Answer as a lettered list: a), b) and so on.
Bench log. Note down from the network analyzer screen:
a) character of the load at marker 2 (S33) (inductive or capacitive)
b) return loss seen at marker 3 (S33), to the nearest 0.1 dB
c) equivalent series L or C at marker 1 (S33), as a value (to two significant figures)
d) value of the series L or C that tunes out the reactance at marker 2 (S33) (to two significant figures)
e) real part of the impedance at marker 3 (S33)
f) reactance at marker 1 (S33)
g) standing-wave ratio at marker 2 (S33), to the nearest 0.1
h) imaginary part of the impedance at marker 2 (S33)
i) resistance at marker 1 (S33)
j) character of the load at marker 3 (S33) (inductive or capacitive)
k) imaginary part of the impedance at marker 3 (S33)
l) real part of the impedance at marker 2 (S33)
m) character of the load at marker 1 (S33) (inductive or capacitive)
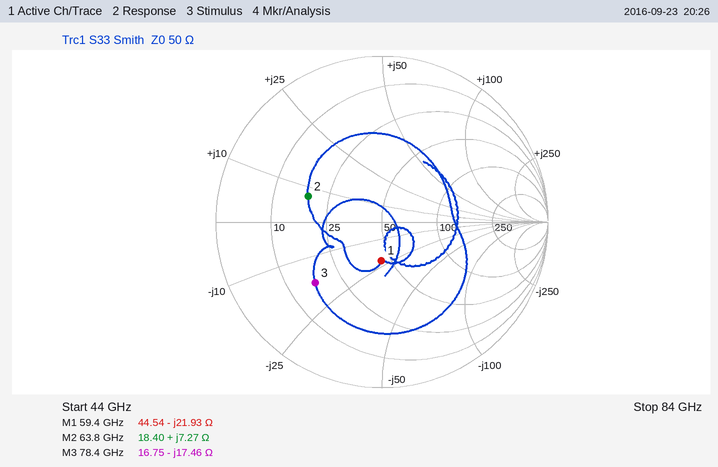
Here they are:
a) inductive
b) 5.3 dB
c) 120 fF
d) 340 fF
e) 16.75 Ω
f) -21.93 Ω
g) 2.8
h) +7.27 Ω
i) 44.54 Ω
j) capacitive
k) -17.46 Ω
l) 18.40 Ω
m) capacitive
